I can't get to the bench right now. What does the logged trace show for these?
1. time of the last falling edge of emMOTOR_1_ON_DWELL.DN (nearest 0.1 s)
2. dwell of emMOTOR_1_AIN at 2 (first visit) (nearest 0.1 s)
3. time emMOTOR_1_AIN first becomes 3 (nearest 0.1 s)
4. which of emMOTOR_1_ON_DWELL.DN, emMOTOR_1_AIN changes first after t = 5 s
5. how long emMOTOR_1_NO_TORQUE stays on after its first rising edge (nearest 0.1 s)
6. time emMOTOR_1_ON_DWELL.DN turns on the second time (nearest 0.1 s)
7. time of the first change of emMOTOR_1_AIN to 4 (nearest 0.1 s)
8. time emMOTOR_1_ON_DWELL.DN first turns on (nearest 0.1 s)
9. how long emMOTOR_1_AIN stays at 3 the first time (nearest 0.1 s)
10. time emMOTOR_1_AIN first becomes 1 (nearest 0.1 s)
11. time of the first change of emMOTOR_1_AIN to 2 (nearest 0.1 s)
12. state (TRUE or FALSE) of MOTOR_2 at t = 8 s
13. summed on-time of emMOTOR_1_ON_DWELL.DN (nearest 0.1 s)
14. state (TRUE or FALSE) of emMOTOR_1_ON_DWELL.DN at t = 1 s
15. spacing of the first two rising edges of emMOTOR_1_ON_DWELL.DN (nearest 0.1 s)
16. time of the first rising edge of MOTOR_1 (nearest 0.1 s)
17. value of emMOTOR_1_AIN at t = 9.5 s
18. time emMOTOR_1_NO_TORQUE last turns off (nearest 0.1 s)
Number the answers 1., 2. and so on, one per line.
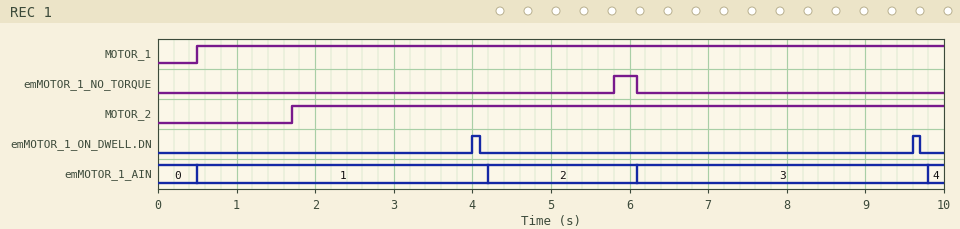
1. 9.7 s
2. 1.9 s
3. 6.1 s
4. emMOTOR_1_AIN
5. 0.3 s
6. 9.6 s
7. 9.8 s
8. 4.0 s
9. 3.7 s
10. 0.5 s
11. 4.2 s
12. TRUE
13. 0.2 s
14. FALSE
15. 5.6 s
16. 0.5 s
17. 3
18. 6.1 s
